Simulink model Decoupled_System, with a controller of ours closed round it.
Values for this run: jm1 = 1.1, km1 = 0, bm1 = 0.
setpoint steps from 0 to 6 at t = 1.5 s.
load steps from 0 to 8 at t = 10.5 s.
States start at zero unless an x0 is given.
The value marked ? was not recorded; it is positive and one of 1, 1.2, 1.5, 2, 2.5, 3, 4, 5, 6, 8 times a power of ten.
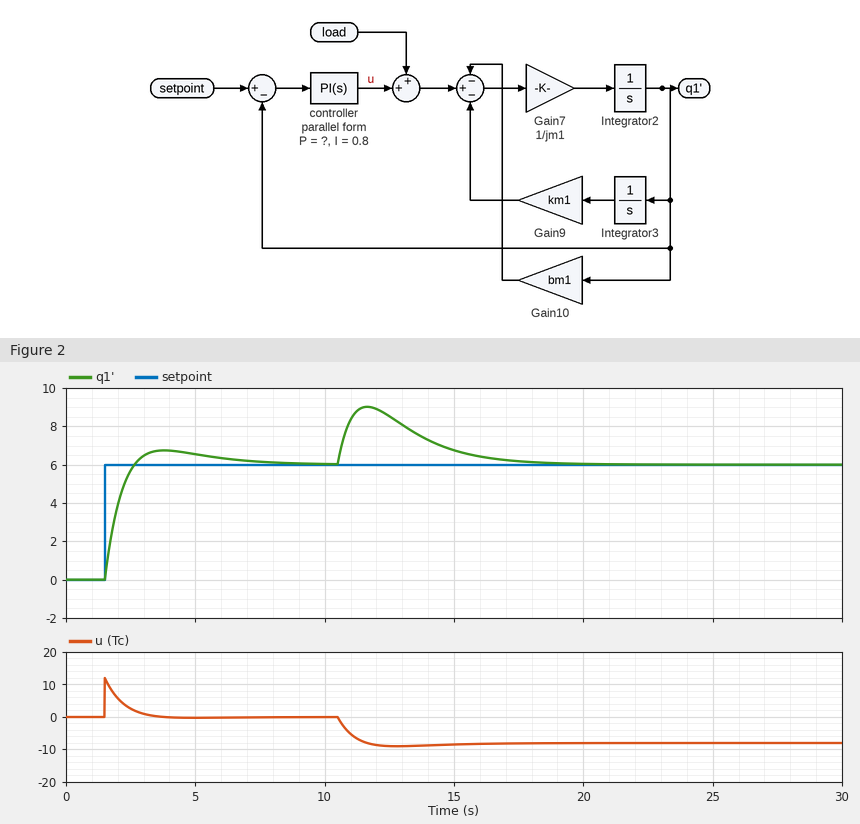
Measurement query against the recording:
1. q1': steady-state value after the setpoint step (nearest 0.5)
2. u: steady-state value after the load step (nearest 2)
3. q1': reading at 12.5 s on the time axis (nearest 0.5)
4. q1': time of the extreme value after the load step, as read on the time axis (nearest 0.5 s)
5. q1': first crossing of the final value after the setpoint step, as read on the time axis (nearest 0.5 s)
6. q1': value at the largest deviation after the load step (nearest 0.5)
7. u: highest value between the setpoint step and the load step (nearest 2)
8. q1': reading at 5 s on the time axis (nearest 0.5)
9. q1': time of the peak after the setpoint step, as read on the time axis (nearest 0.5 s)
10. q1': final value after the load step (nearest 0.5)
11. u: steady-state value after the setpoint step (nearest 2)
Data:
6.0
-8
8.5
11.5 s
2.5 s
9.0
12
6.5
4.0 s
6.0
0
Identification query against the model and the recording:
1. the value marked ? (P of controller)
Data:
2
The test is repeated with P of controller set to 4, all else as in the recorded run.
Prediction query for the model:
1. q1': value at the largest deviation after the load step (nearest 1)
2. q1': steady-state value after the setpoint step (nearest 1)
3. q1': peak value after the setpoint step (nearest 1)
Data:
8
6
6
